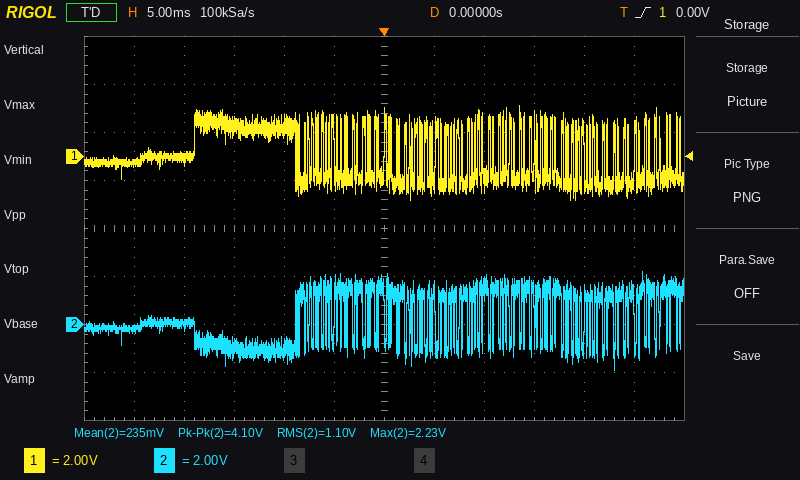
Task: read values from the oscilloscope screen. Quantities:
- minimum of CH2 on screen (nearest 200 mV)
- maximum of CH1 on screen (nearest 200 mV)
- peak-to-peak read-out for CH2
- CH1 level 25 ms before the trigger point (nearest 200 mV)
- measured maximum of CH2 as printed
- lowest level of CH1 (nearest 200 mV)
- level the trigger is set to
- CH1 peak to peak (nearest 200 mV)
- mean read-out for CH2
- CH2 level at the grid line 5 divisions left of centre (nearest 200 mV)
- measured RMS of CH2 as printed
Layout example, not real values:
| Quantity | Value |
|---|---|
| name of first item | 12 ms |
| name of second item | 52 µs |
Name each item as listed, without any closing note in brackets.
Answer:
| Quantity | Value |
|---|---|
| minimum of CH2 on screen | -1.8 V |
| maximum of CH1 on screen | 2.2 V |
| peak-to-peak read-out for CH2 | 4.10 V |
| CH1 level 25 ms before the trigger point | -200 mV |
| measured maximum of CH2 as printed | 2.23 V |
| lowest level of CH1 | -1.8 V |
| level the trigger is set to | 0.00 V |
| CH1 peak to peak | 4.0 V |
| mean read-out for CH2 | 235 mV |
| CH2 level at the grid line 5 divisions left of centre | -200 mV |
| measured RMS of CH2 as printed | 1.10 V |
